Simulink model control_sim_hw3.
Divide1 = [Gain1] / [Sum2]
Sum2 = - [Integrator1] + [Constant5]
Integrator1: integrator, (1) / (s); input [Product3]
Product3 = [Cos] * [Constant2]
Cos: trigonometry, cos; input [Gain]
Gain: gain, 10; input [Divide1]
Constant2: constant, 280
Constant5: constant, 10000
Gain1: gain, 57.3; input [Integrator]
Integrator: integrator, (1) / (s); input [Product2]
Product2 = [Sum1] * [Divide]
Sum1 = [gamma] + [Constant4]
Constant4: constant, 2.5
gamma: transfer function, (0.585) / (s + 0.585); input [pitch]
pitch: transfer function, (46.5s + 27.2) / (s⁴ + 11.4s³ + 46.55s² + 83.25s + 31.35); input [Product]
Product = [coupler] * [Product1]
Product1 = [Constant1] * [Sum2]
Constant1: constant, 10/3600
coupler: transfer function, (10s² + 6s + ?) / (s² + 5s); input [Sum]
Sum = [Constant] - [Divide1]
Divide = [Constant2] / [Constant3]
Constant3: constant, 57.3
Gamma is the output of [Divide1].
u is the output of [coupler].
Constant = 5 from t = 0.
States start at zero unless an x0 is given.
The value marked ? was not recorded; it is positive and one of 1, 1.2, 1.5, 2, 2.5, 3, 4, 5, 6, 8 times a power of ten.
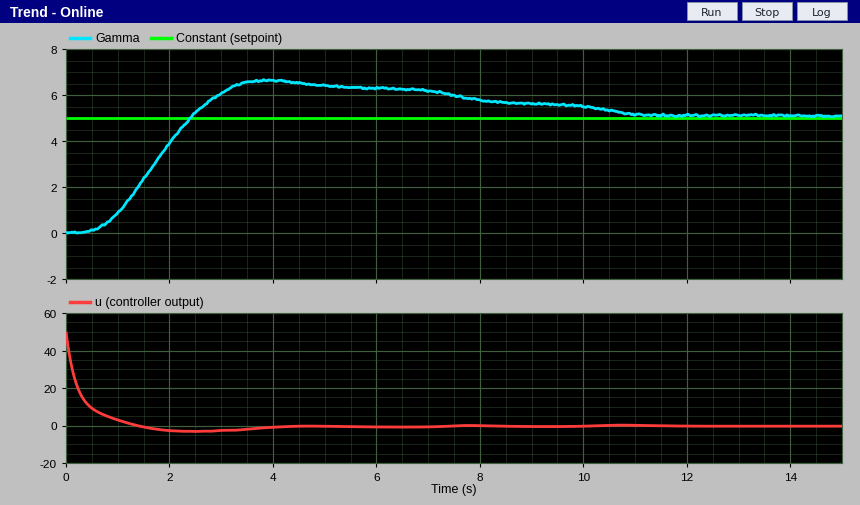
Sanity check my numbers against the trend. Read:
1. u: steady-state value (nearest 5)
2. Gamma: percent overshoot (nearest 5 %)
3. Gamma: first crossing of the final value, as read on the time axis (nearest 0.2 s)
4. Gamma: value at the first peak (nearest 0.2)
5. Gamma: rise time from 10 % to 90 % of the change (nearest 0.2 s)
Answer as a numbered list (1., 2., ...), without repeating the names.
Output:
1. 0
2. 30 %
3. 2.4 s
4. 6.6
5. 1.4 s
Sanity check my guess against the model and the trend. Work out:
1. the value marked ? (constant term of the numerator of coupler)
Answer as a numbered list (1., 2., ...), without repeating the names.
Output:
1. 1
